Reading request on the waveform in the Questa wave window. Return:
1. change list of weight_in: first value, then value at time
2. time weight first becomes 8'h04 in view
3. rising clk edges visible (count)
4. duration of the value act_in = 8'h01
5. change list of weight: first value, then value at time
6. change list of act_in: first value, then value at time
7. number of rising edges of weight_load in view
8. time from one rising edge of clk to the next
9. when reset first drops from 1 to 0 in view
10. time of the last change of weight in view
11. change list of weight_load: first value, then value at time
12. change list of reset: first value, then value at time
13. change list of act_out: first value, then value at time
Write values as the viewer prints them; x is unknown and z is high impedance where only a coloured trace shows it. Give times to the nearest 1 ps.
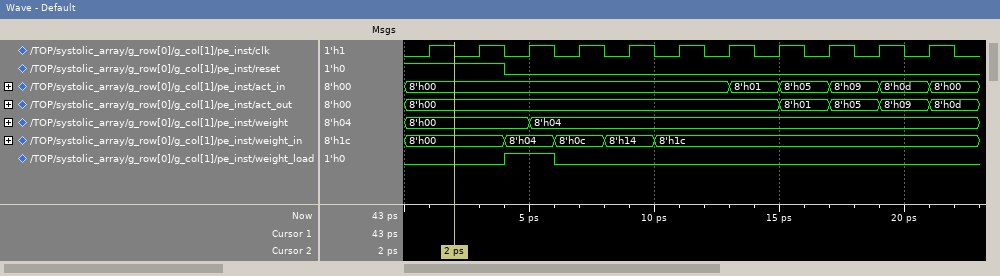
8'h00, 8'h04 at 4 ps, 8'h0c at 6 ps, 8'h14 at 8 ps, 8'h1c at 10 ps
5 ps
11
2 ps
8'h00, 8'h04 at 5 ps
8'h00, 8'h01 at 13 ps, 8'h05 at 15 ps, 8'h09 at 17 ps, 8'h0d at 19 ps, 8'h00 at 21 ps
1
2 ps
4 ps
5 ps
0, 1 at 4 ps, 0 at 6 ps
1, 0 at 4 ps
8'h00, 8'h01 at 15 ps, 8'h05 at 17 ps, 8'h09 at 19 ps, 8'h0d at 21 ps
